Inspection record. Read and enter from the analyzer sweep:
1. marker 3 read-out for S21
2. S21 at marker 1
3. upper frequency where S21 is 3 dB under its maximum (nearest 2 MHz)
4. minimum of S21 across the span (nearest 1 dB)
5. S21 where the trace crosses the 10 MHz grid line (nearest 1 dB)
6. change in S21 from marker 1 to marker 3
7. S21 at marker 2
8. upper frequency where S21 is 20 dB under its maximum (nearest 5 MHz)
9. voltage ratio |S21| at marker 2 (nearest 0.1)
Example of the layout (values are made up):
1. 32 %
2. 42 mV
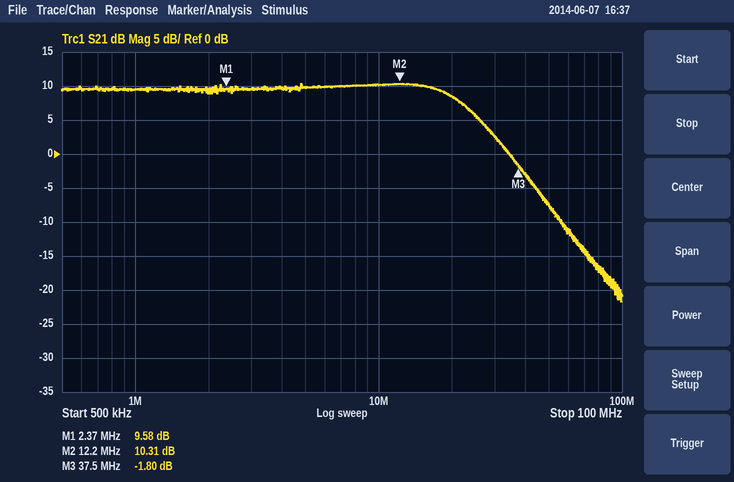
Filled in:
1. -1.80 dB
2. 9.58 dB
3. 22 MHz
4. -22 dB
5. 10 dB
6. -11.38 dB
7. 10.31 dB
8. 55 MHz
9. 3.3
